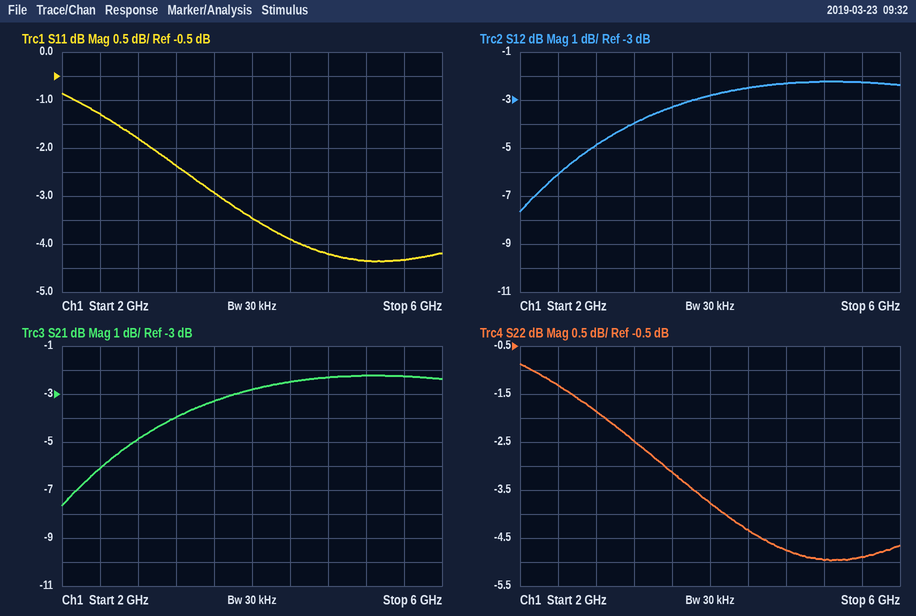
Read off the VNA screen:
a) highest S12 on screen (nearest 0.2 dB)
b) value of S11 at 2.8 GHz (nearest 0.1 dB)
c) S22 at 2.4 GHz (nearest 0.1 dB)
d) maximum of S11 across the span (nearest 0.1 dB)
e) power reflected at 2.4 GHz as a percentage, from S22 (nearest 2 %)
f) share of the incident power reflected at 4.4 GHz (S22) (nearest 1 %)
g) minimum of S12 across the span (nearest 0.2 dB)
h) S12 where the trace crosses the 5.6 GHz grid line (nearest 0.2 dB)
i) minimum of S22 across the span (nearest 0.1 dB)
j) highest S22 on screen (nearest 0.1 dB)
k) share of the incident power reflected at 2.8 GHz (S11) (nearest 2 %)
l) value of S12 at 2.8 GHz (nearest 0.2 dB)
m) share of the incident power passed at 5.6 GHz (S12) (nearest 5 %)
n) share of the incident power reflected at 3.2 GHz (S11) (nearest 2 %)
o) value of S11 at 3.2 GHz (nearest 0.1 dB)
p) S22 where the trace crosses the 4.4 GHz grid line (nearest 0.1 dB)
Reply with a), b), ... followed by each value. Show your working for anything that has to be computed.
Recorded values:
a) -2.2 dB
b) -1.8 dB
c) -1.3 dB
d) -0.9 dB
e) 10^(-1.3/10) ≈ 74 %
f) 10^(-4.3/10) ≈ 37 %
g) -7.6 dB
h) -2.2 dB
i) -5.0 dB
j) -0.9 dB
k) 10^(-1.8/10) ≈ 66 %
l) -4.8 dB
m) 10^(-2.2/10) ≈ 60 %
n) 10^(-2.4/10) ≈ 58 %
o) -2.4 dB
p) -4.3 dB
